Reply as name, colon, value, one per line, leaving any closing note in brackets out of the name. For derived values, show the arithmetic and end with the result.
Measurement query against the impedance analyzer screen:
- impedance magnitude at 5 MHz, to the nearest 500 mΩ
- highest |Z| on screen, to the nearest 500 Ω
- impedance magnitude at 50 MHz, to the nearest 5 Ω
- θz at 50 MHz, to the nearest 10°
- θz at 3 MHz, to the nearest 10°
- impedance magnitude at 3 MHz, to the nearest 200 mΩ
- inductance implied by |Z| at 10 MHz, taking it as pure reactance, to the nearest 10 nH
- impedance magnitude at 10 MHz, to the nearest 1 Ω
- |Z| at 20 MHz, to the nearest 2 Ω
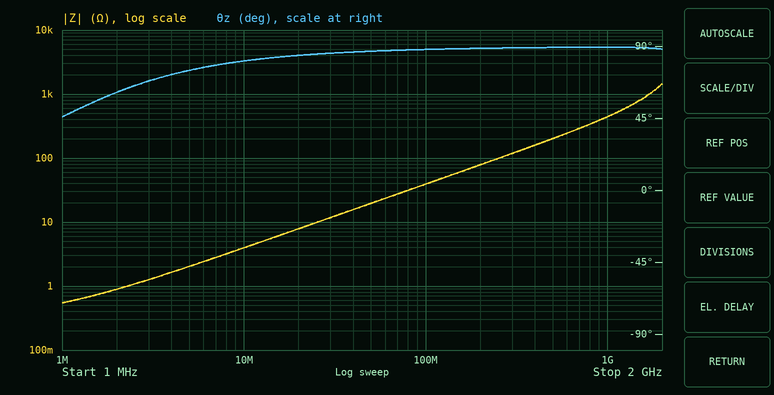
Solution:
impedance magnitude at 5 MHz, to the nearest 500 mΩ: 2.0 Ω
highest |Z| on screen, to the nearest 500 Ω: 1.5 kΩ
impedance magnitude at 50 MHz, to the nearest 5 Ω: 20 Ω
θz at 50 MHz, to the nearest 10°: 90°
θz at 3 MHz, to the nearest 10°: 70°
impedance magnitude at 3 MHz, to the nearest 200 mΩ: 1.2 Ω
inductance implied by |Z| at 10 MHz, taking it as pure reactance, to the nearest 10 nH: L = 4 Ω/(2π × 10 MHz) ≈ 63.7 nH, so 60 nH to the nearest 10 nH
impedance magnitude at 10 MHz, to the nearest 1 Ω: 4 Ω
|Z| at 20 MHz, to the nearest 2 Ω: 8 Ω
